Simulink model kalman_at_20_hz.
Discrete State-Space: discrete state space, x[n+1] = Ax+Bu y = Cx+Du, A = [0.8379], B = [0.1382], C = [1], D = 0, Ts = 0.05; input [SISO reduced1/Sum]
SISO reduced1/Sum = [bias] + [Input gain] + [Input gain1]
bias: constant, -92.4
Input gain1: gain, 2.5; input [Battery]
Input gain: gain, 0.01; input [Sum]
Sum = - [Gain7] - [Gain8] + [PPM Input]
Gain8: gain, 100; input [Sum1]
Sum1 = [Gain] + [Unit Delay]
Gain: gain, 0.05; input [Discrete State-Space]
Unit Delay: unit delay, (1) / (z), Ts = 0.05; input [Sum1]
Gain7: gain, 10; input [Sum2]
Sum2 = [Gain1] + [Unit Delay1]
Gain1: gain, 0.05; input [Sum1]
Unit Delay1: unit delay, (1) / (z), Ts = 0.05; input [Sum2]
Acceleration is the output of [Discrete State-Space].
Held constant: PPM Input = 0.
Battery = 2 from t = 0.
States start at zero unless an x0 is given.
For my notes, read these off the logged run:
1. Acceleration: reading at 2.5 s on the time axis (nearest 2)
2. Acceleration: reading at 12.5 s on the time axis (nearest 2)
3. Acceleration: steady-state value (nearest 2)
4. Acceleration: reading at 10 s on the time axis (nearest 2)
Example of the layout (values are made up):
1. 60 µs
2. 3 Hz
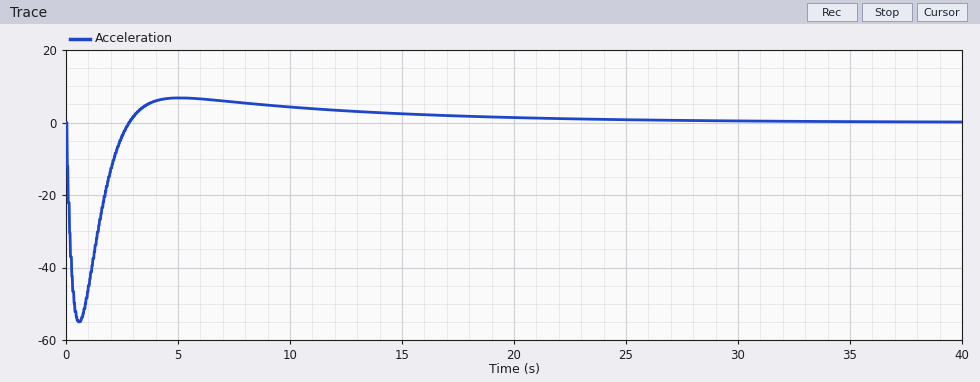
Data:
1. -4
2. 4
3. 0
4. 4
